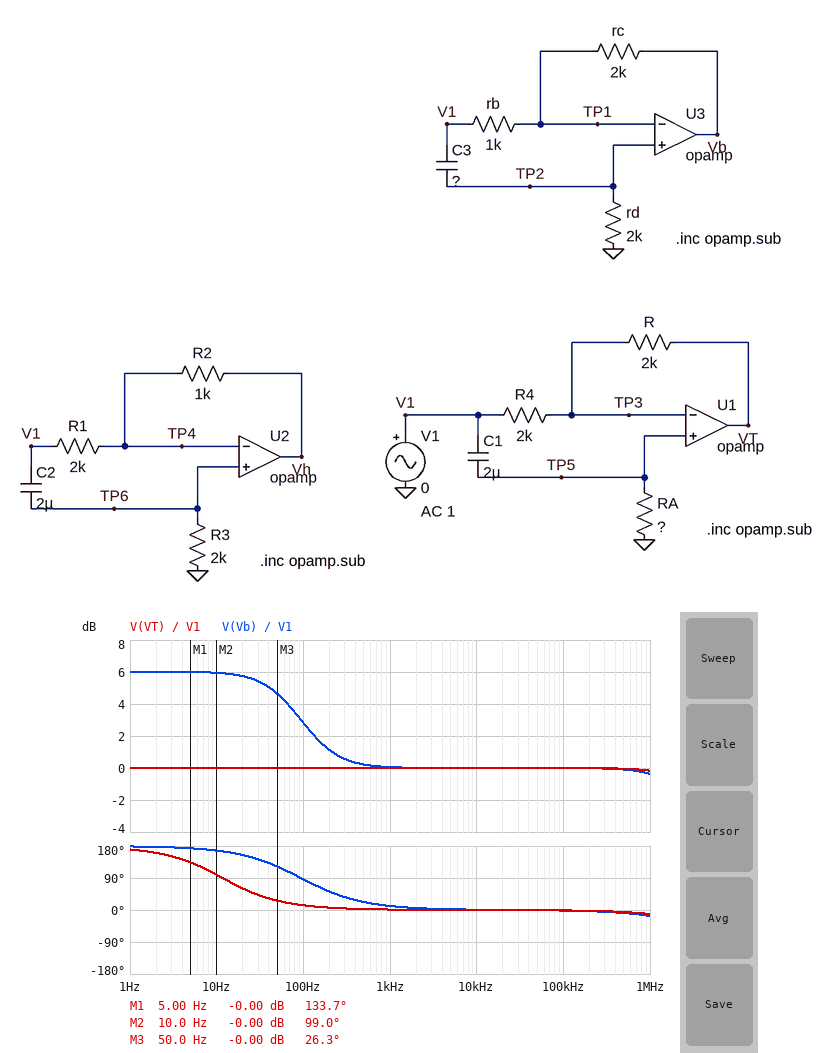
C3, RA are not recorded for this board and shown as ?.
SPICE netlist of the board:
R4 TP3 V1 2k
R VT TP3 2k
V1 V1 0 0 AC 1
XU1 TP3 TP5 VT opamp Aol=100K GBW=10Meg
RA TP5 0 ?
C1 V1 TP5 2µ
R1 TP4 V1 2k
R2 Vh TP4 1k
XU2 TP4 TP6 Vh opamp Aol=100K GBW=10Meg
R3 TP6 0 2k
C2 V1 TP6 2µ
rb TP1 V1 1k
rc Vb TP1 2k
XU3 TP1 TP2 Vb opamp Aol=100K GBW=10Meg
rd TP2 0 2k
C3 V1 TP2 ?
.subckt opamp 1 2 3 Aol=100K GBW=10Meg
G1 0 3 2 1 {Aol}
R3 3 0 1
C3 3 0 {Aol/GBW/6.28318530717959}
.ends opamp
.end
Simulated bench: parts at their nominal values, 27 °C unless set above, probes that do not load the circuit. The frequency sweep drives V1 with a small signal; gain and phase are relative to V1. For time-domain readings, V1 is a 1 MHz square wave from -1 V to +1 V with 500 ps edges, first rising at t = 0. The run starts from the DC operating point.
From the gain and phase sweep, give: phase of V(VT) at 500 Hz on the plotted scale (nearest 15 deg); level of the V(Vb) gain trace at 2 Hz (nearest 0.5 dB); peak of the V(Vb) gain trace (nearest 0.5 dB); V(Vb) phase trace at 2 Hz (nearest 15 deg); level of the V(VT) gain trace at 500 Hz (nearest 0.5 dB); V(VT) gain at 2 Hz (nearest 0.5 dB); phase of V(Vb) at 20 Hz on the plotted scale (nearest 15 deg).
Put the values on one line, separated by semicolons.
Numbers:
0 deg; 6.0 dB; 6.0 dB; 180 deg; 0 dB; 0 dB; 150 deg
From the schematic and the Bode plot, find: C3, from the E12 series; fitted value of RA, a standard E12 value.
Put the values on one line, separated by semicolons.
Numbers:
1.2 µF; 6.8 kΩ
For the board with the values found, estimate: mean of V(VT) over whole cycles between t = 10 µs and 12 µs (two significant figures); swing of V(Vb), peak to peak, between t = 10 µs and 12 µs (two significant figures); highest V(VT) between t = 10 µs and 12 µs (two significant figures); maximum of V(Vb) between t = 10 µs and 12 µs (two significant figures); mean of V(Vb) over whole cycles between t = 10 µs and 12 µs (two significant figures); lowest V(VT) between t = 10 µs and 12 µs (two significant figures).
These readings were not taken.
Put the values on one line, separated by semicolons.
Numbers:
2.0 V; 2.0 V; 3.0 V; 4.0 V; 3.0 V; 1.0 V
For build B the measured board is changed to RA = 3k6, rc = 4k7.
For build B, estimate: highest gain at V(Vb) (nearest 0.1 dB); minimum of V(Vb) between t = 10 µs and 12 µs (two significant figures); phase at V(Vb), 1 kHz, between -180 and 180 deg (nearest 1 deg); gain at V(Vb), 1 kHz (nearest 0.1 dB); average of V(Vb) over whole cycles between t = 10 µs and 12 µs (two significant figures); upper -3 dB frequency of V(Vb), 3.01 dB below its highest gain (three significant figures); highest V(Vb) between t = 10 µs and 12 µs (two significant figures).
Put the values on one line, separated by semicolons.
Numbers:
13.4 dB; 4.7 V; 21 deg; 0.4 dB; 5.7 V; 69.5 Hz; 6.7 V
